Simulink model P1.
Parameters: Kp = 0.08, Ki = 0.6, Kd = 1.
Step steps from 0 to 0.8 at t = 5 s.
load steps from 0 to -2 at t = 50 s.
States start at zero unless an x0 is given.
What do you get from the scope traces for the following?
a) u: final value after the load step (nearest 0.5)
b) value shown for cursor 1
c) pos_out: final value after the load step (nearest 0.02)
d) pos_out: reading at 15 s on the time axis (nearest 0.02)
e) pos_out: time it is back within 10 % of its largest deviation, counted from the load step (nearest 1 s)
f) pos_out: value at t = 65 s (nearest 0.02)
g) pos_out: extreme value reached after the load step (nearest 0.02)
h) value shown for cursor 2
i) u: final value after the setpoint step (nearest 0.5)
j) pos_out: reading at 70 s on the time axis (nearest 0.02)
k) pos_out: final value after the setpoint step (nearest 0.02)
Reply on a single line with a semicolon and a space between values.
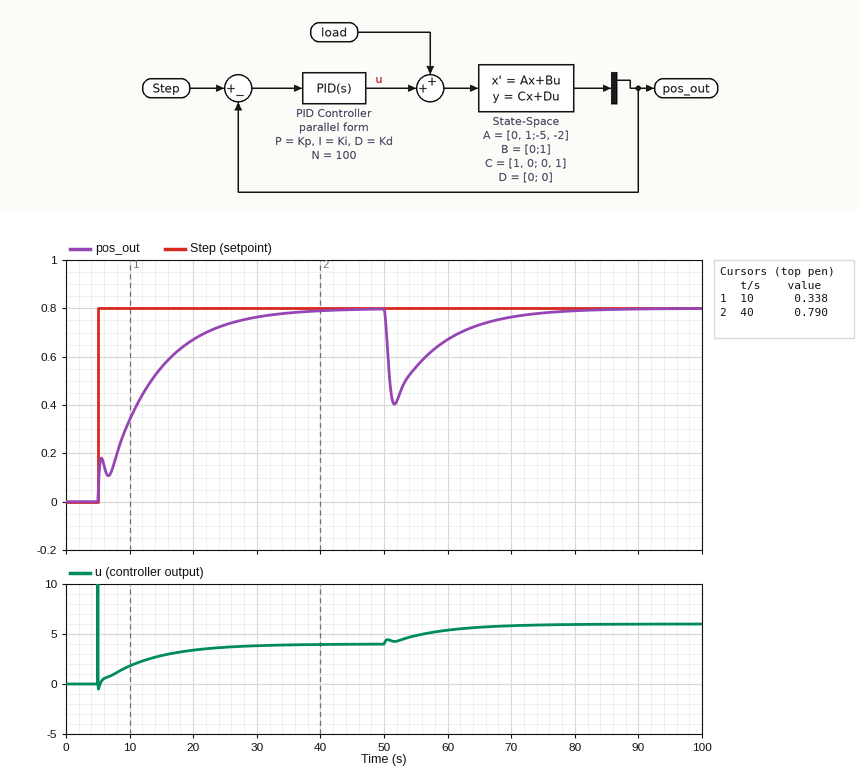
6.0; 0.338; 0.80; 0.56; 19 s; 0.74; 0.40; 0.790; 4.0; 0.76; 0.80
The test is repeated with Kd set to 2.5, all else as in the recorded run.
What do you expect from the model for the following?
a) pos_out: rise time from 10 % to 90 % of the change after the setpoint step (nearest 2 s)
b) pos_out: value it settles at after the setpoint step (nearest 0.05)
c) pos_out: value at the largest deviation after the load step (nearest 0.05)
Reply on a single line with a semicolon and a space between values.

18 s; 0.80; 0.45
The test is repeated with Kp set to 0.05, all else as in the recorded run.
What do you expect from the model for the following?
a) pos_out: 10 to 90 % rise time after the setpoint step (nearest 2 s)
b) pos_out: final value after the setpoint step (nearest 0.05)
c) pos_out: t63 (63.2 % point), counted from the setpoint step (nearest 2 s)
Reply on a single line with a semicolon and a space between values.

18 s; 0.80; 8 s
